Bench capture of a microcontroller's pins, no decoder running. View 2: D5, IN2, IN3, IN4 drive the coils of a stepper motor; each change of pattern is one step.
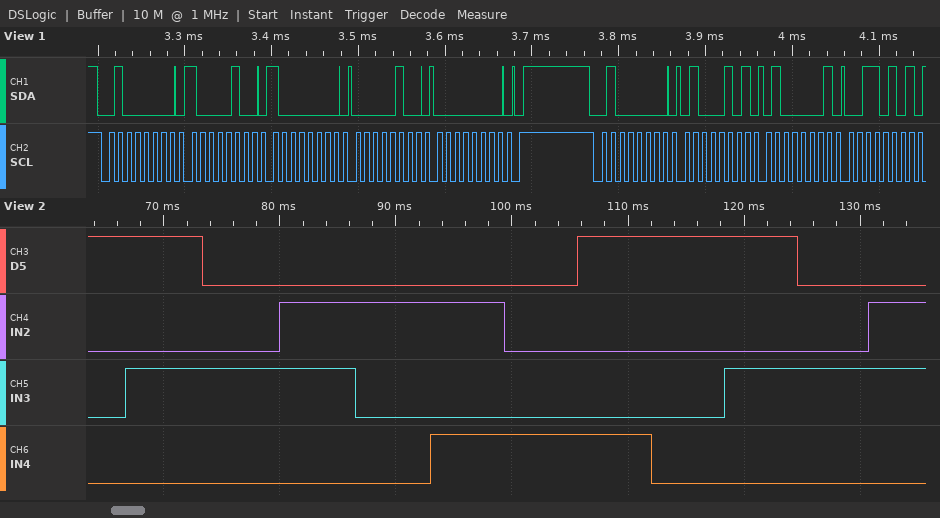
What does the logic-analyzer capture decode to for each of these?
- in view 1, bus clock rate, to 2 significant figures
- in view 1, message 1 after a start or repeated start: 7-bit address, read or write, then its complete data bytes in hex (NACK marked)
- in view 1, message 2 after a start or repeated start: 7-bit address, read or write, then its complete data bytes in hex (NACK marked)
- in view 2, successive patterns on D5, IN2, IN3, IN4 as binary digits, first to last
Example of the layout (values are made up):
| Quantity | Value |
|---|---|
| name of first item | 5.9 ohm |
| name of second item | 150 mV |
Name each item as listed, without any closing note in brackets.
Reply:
| Quantity | Value |
|---|---|
| in view 1, bus clock rate, to 2 significant figures | 100 kHz |
| in view 1, message 1 after a start or repeated start: 7-bit address, read or write, then its complete data bytes in hex | 0x20 write: 84 80 04 00 |
| in view 1, message 2 after a start or repeated start: 7-bit address, read or write, then its complete data bytes in hex | 0x20 write: 45 41 35 |
| in view 2, successive patterns on D5, IN2, IN3, IN4 as binary digits, first to last | 1000 1010 0010 0110 0100 0101 0001 1001 1000 1010 0010 0110 |
